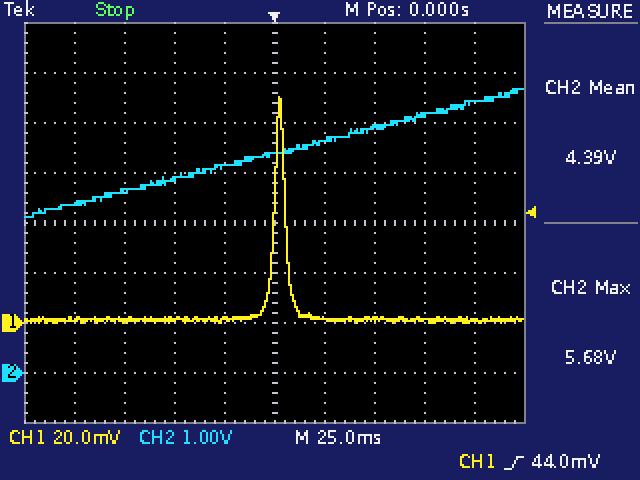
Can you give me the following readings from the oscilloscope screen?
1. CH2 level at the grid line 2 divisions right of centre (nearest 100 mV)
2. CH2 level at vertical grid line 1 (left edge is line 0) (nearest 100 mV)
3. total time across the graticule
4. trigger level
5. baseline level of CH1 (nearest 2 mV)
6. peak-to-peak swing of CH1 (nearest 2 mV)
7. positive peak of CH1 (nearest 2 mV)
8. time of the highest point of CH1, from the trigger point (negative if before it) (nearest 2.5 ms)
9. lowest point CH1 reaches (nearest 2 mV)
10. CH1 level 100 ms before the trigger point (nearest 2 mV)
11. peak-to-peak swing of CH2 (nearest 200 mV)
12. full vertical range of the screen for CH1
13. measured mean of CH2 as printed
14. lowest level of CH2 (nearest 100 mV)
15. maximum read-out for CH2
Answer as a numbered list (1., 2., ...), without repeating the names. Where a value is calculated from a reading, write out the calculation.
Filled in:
1. 4.9 V
2. 3.4 V
3. 250 ms
4. 44.0 mV
5. 2 mV
6. 90 mV − (0 mV) = 90 mV
7. 90 mV
8. +2.5 ms
9. 0 mV
10. 2 mV
11. 2.6 V
12. 160 mV
13. 4.39 V
14. 3.1 V
15. 5.68 V
